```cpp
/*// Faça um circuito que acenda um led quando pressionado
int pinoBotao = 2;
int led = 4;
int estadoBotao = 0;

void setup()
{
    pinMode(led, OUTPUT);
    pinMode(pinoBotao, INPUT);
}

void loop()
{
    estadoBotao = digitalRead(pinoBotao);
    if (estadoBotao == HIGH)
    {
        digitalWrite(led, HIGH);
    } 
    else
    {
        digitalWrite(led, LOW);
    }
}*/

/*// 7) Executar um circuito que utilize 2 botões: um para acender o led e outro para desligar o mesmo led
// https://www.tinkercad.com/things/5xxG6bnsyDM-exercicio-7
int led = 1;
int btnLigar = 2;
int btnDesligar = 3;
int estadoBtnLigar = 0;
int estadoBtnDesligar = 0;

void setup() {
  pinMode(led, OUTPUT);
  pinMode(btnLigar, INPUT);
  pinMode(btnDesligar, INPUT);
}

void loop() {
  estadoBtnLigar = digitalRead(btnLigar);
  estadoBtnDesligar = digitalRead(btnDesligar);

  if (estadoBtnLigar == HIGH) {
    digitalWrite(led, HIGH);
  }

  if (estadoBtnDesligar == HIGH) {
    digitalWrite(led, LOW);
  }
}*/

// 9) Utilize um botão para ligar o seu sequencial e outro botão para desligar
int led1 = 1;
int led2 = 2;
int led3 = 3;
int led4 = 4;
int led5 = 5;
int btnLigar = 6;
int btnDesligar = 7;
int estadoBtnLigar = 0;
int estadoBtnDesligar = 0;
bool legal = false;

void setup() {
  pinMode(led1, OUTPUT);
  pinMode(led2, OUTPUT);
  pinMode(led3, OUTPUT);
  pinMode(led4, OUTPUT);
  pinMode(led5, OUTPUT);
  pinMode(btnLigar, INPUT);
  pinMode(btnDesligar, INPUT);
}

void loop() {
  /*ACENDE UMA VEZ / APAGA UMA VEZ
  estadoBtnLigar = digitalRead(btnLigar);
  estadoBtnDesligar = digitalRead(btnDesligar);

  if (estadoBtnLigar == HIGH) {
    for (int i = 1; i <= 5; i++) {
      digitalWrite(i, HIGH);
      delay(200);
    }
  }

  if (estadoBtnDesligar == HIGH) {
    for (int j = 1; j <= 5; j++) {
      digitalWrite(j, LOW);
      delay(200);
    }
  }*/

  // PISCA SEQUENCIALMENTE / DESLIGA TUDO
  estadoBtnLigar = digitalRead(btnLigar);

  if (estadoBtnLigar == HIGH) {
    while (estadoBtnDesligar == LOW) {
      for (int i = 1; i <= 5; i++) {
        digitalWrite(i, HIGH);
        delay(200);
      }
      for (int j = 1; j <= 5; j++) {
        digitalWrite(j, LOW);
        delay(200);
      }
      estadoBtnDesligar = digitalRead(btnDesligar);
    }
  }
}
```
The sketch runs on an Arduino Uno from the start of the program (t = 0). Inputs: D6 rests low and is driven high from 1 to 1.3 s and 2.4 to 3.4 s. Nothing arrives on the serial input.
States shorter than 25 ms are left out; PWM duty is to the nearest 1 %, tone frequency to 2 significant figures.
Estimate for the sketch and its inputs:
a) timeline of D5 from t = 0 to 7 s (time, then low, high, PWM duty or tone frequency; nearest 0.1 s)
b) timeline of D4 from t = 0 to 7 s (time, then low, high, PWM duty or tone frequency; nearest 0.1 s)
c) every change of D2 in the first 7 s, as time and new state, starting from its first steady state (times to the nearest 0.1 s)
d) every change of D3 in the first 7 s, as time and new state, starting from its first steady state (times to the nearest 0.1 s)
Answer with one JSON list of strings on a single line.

["0 s low; 1.8 s high; 2.8 s low; 3.8 s high; 4.8 s low; 5.8 s high; 6.8 s low", "0 s low; 1.6 s high; 2.6 s low; 3.6 s high; 4.6 s low; 5.6 s high; 6.6 s low", "0 s low; 1.2 s high; 2.2 s low; 3.2 s high; 4.2 s low; 5.2 s high; 6.2 s low", "0 s low; 1.4 s high; 2.4 s low; 3.4 s high; 4.4 s low; 5.4 s high; 6.4 s low"]
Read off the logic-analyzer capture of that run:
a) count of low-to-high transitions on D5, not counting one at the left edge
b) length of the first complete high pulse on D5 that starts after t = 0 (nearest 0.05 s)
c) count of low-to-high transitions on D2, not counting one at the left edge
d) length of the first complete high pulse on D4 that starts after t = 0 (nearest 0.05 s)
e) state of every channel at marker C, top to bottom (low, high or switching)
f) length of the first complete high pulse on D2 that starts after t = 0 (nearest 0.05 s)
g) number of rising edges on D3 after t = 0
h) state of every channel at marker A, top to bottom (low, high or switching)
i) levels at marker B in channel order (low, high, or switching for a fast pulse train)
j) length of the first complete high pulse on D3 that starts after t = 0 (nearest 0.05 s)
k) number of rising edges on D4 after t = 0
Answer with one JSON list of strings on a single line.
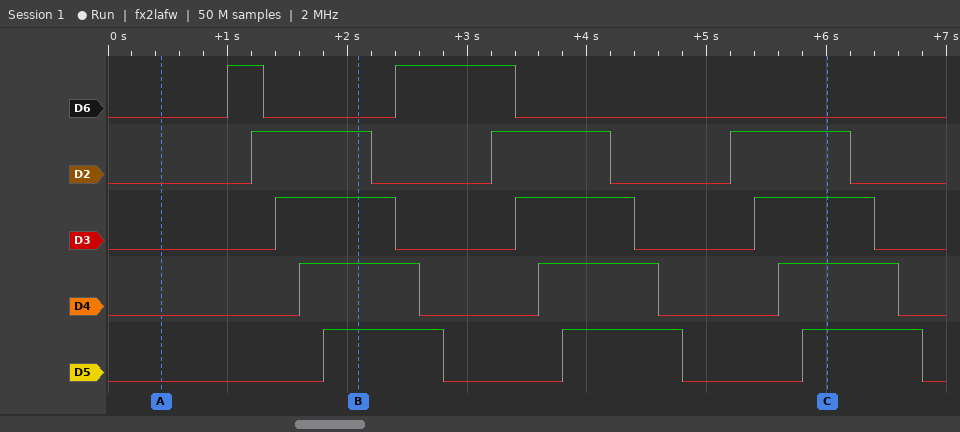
["3", "1.00 s", "3", "1.00 s", "D6 low, D2 high, D3 high, D4 high, D5 high", "1.00 s", "3", "D6 low, D2 low, D3 low, D4 low, D5 low", "D6 low, D2 high, D3 high, D4 high, D5 high", "1.00 s", "3"]
